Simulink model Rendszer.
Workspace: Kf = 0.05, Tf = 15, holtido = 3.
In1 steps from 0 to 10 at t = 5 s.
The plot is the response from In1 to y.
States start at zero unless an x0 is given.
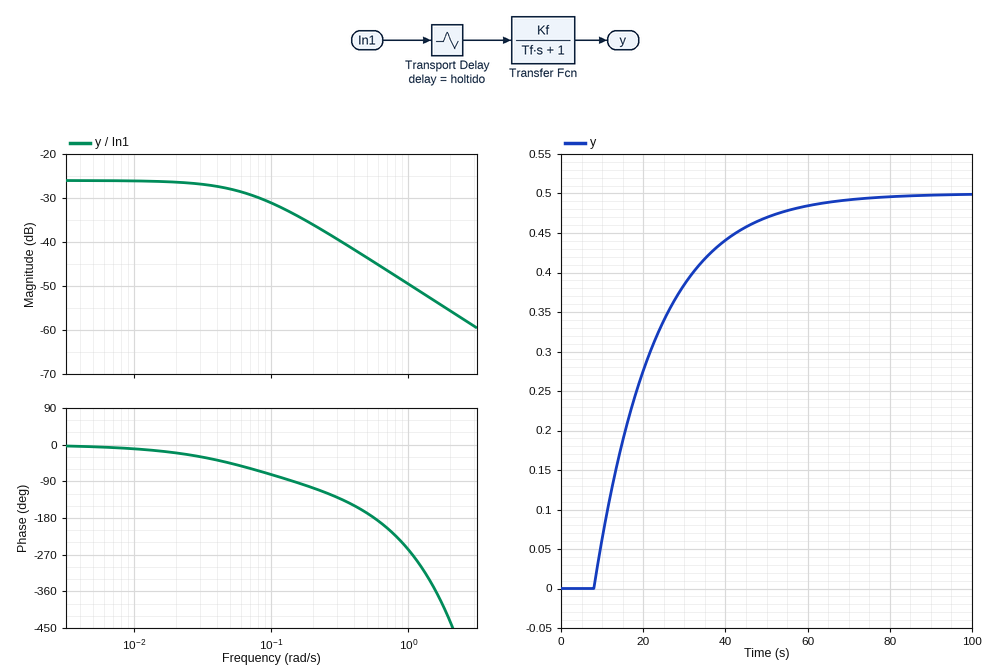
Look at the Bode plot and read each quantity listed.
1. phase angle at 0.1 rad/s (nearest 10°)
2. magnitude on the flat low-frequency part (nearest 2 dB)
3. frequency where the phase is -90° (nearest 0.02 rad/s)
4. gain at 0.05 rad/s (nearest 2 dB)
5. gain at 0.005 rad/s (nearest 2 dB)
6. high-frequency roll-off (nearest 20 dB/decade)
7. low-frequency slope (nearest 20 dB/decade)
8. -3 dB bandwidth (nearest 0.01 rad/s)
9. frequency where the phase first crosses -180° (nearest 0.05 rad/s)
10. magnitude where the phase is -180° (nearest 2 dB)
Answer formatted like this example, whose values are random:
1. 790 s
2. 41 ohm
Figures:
1. -70°
2. -26 dB
3. 0.14 rad/s
4. -28 dB
5. -26 dB
6. -20 dB/decade
7. 0 dB/decade
8. 0.07 rad/s
9. 0.55 rad/s
10. -44 dB
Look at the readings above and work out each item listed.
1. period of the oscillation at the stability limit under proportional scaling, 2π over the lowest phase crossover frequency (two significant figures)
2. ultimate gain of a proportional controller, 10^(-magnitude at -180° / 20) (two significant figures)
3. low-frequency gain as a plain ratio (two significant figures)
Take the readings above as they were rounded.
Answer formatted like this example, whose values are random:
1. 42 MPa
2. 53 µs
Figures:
1. 11 s
2. 160
3. 0.050
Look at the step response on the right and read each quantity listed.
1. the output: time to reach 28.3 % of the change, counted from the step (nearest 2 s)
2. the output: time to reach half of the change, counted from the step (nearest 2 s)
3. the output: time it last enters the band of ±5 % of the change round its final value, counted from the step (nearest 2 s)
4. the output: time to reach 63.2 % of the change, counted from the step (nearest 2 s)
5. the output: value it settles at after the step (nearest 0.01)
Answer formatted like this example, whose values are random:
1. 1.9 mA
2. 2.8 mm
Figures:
1. 8 s
2. 14 s
3. 48 s
4. 18 s
5. 0.50
